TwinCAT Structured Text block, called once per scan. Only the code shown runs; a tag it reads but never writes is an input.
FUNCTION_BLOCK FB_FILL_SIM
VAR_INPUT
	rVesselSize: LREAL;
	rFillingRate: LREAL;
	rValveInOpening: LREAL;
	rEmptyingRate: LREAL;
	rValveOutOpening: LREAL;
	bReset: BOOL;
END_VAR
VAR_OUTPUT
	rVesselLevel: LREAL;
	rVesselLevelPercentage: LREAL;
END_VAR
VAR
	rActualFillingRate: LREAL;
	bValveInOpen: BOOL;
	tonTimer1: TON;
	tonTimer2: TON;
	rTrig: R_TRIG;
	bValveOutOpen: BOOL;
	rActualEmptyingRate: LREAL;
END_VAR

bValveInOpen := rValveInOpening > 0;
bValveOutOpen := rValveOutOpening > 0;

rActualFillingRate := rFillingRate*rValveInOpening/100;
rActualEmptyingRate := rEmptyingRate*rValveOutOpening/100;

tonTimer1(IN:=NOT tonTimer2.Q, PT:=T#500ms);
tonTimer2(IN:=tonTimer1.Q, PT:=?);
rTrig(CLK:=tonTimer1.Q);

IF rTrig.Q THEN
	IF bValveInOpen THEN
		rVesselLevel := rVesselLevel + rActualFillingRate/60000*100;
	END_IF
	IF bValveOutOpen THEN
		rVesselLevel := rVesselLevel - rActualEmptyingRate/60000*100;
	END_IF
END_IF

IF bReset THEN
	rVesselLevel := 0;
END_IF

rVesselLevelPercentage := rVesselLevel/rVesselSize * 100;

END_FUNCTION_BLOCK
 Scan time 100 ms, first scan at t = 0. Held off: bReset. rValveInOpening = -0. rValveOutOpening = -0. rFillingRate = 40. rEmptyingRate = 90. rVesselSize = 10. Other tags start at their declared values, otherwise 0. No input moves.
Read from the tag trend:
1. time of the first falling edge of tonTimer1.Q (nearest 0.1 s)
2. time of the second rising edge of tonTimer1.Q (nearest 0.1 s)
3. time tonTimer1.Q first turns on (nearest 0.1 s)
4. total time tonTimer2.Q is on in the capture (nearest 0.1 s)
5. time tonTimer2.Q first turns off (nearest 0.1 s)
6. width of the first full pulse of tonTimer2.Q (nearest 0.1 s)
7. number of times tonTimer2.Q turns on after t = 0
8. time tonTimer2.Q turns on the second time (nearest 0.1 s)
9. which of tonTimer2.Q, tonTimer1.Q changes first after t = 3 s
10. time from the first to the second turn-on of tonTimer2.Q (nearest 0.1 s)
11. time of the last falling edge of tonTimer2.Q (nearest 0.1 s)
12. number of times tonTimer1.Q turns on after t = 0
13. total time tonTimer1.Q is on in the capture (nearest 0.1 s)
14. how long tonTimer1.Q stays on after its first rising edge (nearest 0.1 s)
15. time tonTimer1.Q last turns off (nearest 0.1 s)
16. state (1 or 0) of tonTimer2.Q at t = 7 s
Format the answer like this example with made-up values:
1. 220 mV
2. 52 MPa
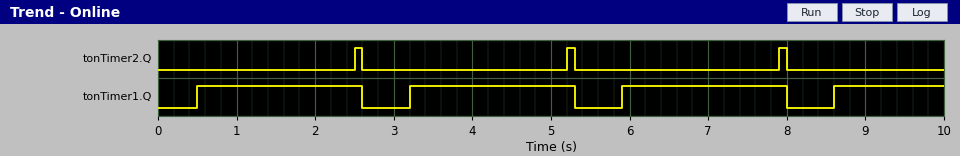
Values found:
1. 2.6 s
2. 3.2 s
3. 0.5 s
4. 0.3 s
5. 2.6 s
6. 0.1 s
7. 3
8. 5.2 s
9. tonTimer1.Q
10. 2.7 s
11. 8.0 s
12. 4
13. 7.7 s
14. 2.1 s
15. 8.0 s
16. 0
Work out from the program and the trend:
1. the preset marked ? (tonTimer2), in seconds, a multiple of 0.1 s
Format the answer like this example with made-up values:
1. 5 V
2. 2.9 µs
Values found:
1. 2.0 s
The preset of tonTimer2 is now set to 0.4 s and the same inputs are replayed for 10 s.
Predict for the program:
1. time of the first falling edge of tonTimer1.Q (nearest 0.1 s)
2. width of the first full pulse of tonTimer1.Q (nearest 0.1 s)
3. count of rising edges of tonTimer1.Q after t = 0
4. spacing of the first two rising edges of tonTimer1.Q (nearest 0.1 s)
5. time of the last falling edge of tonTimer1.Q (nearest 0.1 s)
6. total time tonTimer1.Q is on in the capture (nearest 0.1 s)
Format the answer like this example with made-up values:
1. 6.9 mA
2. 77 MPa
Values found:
1. 1.0 s
2. 0.5 s
3. 9
4. 1.1 s
5. 9.8 s
6. 4.5 s
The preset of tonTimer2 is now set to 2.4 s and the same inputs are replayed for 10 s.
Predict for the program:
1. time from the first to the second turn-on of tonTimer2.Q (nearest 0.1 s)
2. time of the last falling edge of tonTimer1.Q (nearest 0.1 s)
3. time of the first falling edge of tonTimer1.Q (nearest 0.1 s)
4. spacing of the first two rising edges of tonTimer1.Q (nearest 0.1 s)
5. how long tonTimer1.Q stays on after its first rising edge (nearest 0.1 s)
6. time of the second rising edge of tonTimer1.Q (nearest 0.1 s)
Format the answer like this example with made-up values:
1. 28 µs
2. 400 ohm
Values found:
1. 3.1 s
2. 9.2 s
3. 3.0 s
4. 3.1 s
5. 2.5 s
6. 3.6 s
